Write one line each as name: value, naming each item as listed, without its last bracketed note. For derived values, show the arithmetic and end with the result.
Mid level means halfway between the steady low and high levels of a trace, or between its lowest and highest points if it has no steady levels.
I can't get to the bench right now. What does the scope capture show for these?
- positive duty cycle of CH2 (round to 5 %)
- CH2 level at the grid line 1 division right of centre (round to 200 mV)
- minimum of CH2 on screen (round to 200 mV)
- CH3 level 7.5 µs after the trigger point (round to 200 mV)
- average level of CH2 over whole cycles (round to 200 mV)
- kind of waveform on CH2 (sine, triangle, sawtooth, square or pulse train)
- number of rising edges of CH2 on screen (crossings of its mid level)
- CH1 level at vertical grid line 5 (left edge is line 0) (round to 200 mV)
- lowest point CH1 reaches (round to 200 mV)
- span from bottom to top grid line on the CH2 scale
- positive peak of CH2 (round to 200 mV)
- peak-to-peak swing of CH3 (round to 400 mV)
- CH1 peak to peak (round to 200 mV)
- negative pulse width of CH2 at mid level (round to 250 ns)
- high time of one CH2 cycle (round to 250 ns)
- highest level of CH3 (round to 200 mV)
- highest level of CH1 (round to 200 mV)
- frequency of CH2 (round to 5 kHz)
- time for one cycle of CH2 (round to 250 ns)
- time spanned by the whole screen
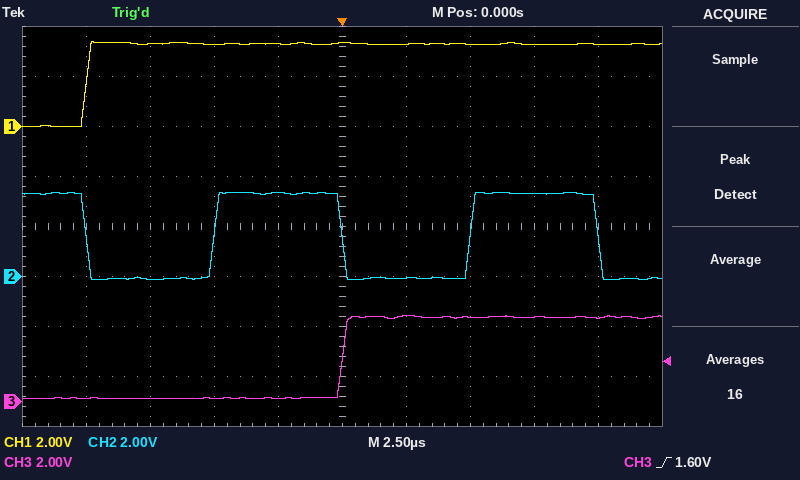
positive duty cycle of CH2: 5.00 µs / 10.00 µs ≈ 50 %
CH2 level at the grid line 1 division right of centre: 0.0 V
minimum of CH2 on screen: -200 mV
CH3 level 7.5 µs after the trigger point: 3.4 V
average level of CH2 over whole cycles: -200 mV + 0.5 × (3.4 V − (-200 mV)) ≈ 1.6 V
kind of waveform on CH2: square
number of rising edges of CH2 on screen: 2
CH1 level at vertical grid line 5 (left edge is line 0): 3.4 V
lowest point CH1 reaches: 0.0 V
span from bottom to top grid line on the CH2 scale: 16 V
positive peak of CH2: 3.4 V
peak-to-peak swing of CH3: 3.2 V
CH1 peak to peak: 3.4 V − (0.0 V) = 3.4 V
negative pulse width of CH2 at mid level: 5.00 µs
high time of one CH2 cycle: 5.00 µs
highest level of CH3: 3.4 V
highest level of CH1: 3.4 V
frequency of CH2: 1 / 10.00 µs ≈ 100 kHz
time for one cycle of CH2: 10.00 µs
time spanned by the whole screen: 25 µs
